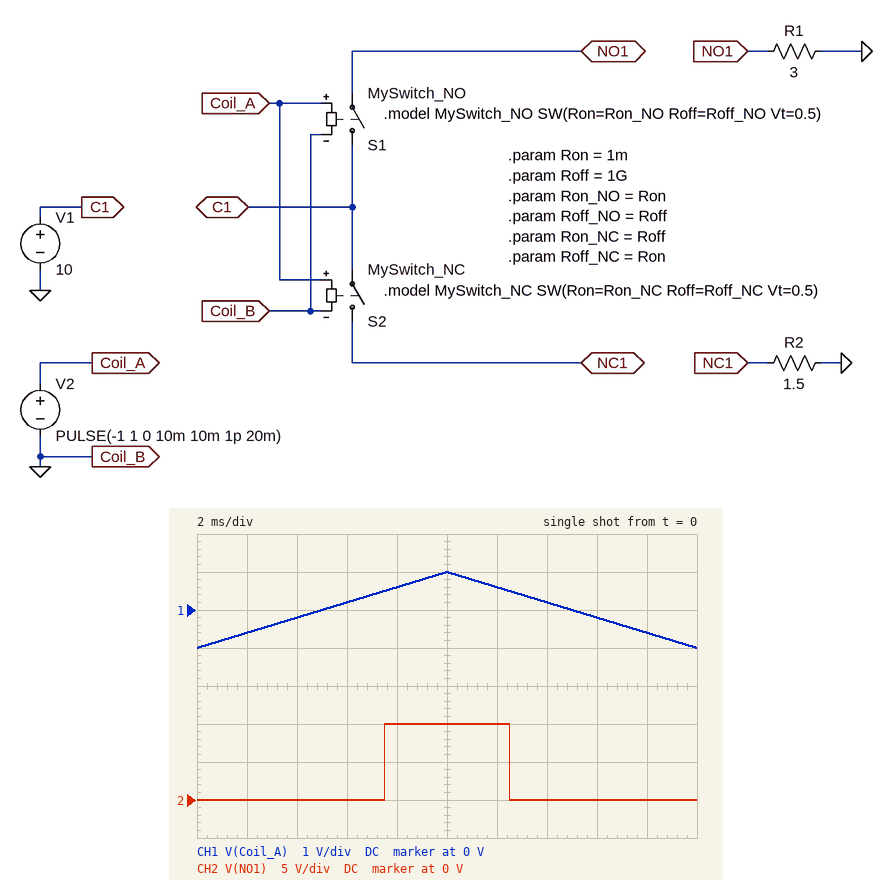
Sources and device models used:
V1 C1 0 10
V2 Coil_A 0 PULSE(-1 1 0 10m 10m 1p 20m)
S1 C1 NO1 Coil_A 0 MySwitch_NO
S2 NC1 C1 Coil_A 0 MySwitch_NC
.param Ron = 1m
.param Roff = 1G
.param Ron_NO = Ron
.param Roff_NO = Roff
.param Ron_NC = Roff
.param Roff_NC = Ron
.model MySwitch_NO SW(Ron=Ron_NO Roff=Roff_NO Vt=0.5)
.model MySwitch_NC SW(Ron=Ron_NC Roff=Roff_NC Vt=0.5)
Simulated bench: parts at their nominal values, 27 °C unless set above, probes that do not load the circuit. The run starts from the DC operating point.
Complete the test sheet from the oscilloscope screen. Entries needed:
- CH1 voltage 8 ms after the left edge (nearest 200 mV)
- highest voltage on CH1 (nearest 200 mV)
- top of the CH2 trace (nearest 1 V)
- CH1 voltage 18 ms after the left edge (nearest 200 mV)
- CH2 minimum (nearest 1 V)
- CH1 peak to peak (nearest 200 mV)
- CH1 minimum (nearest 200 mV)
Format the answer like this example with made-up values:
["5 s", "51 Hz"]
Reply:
["600 mV", "1.0 V", "10 V", "-600 mV", "0 V", "2.0 V", "-1.0 V"]
